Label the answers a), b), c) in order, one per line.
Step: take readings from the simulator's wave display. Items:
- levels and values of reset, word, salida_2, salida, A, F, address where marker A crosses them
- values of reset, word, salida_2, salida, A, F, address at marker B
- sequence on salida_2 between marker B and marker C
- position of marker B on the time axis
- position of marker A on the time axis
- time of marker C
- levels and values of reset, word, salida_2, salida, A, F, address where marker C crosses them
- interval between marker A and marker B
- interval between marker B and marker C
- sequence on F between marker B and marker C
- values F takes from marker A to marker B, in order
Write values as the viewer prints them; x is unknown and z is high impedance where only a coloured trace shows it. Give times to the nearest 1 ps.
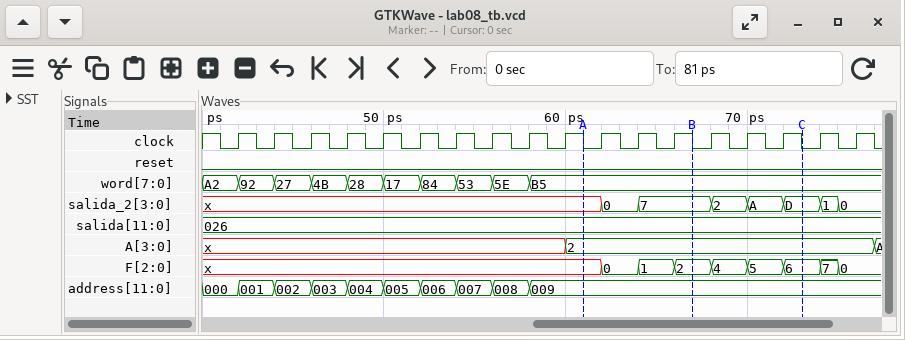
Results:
a) reset=0, word=B5, salida_2=x, salida=026, A=2, F=x, address=009
b) reset=0, word=B5, salida_2=7, salida=026, A=2, F=2, address=009
c) 7, 2, A, D
d) 67 ps
e) 61 ps
f) 73 ps
g) reset=0, word=B5, salida_2=D, salida=026, A=2, F=6, address=009
h) 6 ps
i) 6 ps
j) 2, 4, 5, 6
k) x, 0, 1, 2
